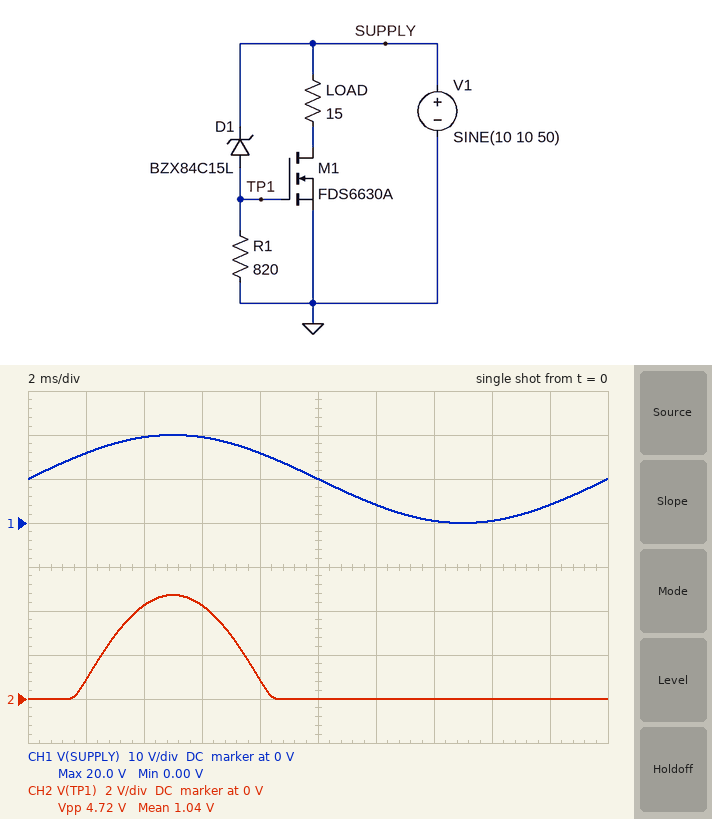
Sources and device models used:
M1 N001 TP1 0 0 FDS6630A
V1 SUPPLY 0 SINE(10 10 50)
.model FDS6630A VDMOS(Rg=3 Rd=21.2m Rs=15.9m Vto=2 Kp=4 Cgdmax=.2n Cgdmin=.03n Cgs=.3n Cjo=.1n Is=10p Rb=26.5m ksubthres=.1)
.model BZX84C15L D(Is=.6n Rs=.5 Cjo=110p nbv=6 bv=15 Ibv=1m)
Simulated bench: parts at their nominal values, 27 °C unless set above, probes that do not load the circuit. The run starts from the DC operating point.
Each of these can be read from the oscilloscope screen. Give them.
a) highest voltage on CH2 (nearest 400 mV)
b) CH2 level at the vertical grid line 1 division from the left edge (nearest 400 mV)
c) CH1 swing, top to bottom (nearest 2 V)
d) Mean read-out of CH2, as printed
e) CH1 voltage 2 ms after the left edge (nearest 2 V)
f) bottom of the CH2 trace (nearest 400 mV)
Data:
4.8 V
800 mV
20 V
1.04 V
16 V
0 V
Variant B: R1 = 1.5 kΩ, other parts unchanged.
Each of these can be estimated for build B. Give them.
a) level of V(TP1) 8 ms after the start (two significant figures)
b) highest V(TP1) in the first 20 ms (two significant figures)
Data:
950 mV
4.8 V
